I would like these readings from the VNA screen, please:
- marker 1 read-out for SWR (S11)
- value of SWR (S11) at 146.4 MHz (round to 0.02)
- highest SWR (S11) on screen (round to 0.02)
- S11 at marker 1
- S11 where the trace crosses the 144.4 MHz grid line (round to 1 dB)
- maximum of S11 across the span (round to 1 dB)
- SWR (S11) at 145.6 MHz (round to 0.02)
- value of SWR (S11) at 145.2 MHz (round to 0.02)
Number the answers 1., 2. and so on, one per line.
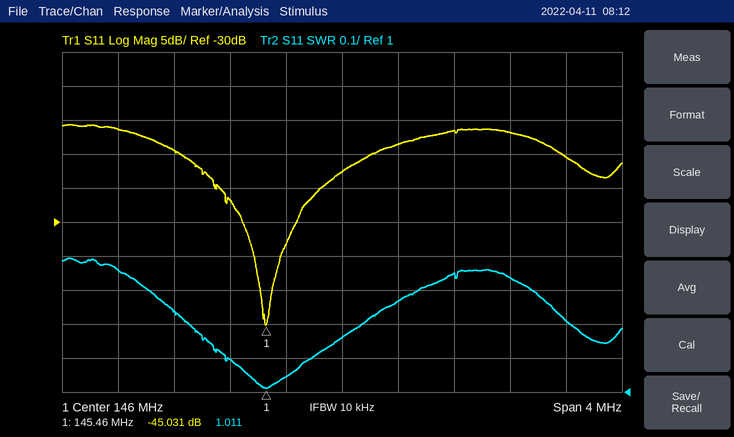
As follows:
1. 1.011
2. 1.26
3. 1.40
4. -45.031 dB
5. -16 dB
6. -16 dB
7. 1.04
8. 1.10
